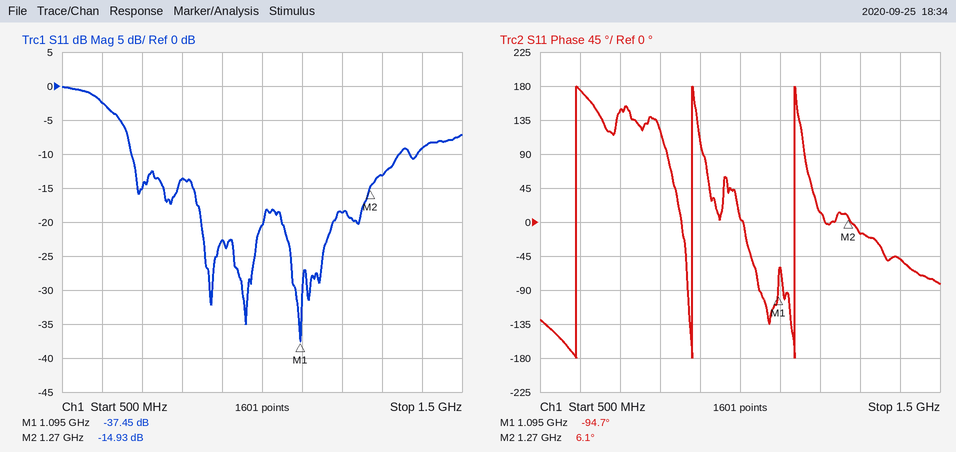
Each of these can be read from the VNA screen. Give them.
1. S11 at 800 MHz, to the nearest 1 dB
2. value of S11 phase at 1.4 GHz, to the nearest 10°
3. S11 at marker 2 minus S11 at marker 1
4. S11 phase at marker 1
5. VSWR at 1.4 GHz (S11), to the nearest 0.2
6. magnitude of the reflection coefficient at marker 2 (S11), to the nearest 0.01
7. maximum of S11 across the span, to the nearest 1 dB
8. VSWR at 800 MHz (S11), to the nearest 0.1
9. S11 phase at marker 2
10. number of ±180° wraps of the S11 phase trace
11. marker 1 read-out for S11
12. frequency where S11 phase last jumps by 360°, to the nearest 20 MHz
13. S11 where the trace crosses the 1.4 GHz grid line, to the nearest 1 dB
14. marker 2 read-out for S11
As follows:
-14 dB
-50°
22.52 dB
-94.7°
2.0
0.18
0 dB
1.5
6.1°
3
-37.45 dB
1.14 GHz
-9 dB
-14.93 dB
